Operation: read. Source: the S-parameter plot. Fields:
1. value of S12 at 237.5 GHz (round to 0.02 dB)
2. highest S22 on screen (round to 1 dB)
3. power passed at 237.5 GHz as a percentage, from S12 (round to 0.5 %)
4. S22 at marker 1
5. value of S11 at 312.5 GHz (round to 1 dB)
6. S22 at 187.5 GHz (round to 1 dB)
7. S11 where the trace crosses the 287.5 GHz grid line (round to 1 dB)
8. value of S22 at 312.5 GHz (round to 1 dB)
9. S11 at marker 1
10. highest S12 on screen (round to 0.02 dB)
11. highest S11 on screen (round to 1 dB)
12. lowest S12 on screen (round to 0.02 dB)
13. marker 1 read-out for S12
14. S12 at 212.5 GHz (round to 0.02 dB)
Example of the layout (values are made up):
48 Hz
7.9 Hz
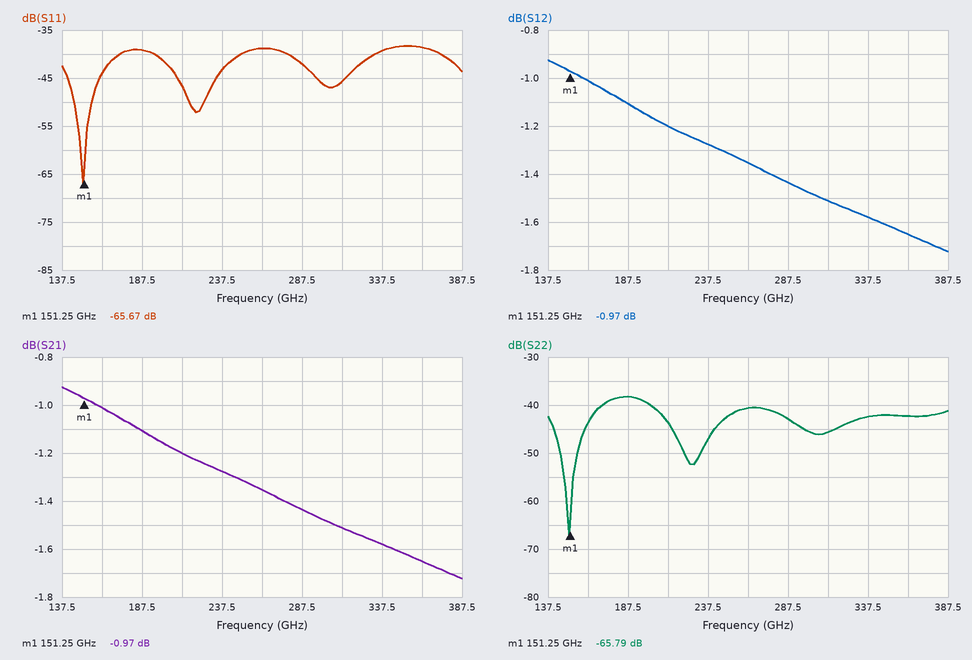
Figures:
-1.28 dB
-38 dB
74.5 %
-65.79 dB
-46 dB
-38 dB
-42 dB
-46 dB
-65.67 dB
-0.92 dB
-38 dB
-1.72 dB
-0.97 dB
-1.20 dB
